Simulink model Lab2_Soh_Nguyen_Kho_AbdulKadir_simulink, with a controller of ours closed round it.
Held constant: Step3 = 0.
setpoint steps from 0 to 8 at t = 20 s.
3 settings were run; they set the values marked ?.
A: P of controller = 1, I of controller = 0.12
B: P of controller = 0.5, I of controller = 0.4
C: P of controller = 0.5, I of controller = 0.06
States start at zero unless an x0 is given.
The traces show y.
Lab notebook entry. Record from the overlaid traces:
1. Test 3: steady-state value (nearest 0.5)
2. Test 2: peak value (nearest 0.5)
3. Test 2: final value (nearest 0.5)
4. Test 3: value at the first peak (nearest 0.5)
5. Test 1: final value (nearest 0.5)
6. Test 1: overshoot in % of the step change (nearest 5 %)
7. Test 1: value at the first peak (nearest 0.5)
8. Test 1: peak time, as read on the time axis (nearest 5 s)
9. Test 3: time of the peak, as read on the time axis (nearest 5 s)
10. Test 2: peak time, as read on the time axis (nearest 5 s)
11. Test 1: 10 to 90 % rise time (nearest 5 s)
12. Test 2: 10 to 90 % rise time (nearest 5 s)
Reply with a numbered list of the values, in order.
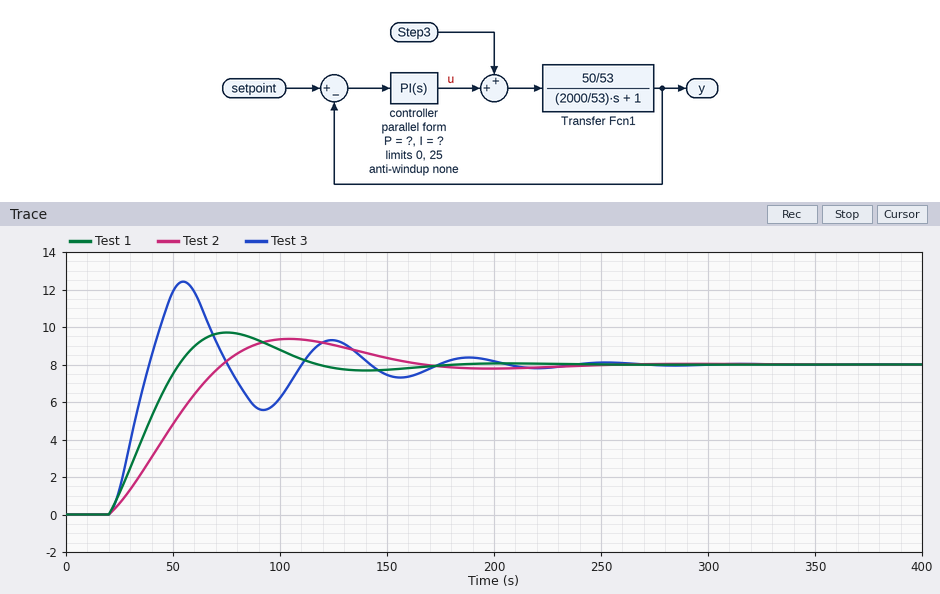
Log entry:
1. 8.0
2. 9.5
3. 8.0
4. 12.5
5. 8.0
6. 20 %
7. 9.5
8. 75 s
9. 55 s
10. 105 s
11. 25 s
12. 40 s
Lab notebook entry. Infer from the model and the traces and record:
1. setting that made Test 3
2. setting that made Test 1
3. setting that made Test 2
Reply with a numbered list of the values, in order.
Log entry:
1. B
2. A
3. C
